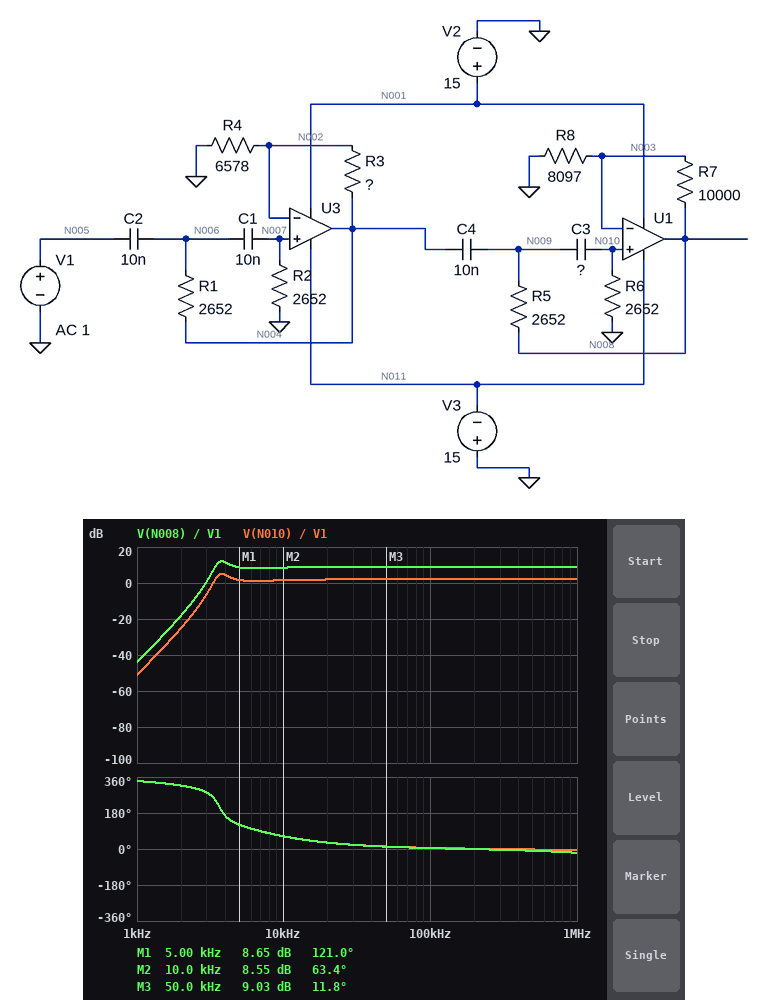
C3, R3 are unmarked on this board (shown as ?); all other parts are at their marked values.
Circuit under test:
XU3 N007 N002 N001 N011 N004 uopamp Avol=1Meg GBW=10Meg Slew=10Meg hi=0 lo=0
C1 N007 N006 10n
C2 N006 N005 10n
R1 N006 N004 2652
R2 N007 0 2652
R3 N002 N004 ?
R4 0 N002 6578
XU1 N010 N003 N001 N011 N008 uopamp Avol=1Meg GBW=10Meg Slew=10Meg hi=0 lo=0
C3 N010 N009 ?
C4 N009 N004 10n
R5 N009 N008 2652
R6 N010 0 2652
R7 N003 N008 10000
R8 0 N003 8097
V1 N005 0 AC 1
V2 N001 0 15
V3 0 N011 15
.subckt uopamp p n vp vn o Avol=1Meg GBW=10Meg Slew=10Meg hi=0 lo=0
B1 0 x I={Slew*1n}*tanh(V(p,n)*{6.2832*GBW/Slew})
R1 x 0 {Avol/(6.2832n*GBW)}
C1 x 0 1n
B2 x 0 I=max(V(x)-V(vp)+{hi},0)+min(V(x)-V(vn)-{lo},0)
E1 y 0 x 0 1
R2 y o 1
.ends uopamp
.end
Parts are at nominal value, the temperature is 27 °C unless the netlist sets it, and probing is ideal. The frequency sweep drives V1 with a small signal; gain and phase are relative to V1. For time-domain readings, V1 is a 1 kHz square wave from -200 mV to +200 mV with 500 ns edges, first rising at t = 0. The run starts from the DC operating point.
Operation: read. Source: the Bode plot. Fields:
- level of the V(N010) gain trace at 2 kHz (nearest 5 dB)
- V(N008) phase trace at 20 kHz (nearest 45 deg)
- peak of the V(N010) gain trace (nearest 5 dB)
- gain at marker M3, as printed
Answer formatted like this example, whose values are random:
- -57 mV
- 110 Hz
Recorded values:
- -25 dB
- 45 deg
- 5 dB
- 9.03 dB
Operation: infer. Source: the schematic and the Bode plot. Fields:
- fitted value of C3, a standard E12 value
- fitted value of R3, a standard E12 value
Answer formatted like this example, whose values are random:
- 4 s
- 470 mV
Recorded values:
- 27 nF
- 1.8 kΩ
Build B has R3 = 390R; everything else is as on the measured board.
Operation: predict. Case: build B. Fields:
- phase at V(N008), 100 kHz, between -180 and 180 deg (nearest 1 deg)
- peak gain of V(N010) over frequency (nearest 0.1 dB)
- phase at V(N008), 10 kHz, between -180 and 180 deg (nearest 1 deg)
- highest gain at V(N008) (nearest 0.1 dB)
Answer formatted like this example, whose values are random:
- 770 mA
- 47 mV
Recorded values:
- 5 deg
- 2.7 dB
- 66 deg
- 9.7 dB
